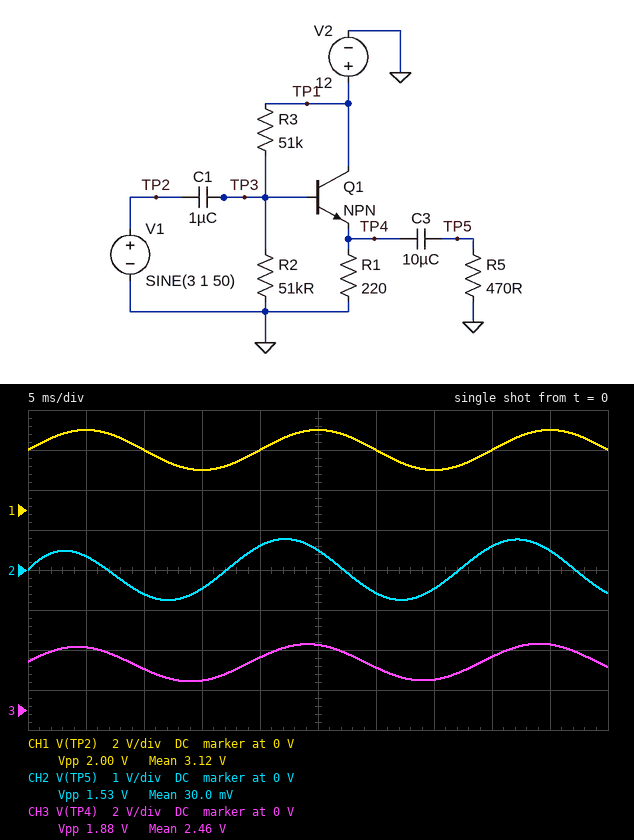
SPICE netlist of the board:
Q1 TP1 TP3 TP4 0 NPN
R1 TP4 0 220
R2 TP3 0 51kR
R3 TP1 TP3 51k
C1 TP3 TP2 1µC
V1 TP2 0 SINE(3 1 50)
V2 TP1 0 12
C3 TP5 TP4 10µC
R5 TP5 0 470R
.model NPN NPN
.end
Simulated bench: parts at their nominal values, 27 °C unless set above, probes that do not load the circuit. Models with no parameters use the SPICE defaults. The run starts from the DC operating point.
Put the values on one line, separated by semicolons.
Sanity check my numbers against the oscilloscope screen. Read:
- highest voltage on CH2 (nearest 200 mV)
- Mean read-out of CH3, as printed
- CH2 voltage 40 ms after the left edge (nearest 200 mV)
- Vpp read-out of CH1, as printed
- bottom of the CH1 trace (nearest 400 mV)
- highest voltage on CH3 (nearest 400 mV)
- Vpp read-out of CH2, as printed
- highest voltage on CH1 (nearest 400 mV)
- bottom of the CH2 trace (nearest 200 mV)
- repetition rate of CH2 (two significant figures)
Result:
800 mV; 2.46 V; 600 mV; 2.00 V; 2.0 V; 3.2 V; 1.53 V; 4.0 V; -800 mV; 50 Hz
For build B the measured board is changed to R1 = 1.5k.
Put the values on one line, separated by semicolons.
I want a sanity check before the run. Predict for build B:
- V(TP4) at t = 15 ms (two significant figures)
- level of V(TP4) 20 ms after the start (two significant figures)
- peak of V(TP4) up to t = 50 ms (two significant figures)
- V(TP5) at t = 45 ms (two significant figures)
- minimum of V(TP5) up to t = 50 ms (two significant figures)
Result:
3.5 V; 4.6 V; 5.4 V; 560 mV; -780 mV
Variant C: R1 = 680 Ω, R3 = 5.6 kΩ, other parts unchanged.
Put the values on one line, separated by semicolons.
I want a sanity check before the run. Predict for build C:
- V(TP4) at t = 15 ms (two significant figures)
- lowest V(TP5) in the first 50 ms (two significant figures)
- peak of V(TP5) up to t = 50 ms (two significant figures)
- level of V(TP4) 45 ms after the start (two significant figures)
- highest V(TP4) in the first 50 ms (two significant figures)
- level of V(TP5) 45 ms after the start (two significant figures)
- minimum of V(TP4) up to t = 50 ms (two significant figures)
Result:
8.6 V; -650 mV; 670 mV; 9.9 V; 10 V; 230 mV; 8.5 V
